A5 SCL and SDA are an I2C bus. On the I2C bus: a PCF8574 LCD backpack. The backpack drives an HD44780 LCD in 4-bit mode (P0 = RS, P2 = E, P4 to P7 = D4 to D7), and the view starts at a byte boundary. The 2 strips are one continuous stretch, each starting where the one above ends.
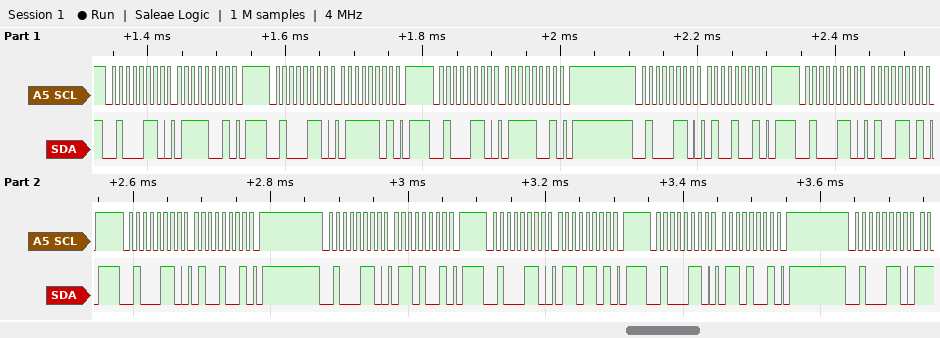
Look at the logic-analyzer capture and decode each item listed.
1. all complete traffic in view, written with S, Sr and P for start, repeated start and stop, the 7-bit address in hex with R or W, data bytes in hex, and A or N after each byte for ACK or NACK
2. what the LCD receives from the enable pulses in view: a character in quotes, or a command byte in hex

S 23W A 79 A P S 23W A 7D A P S 23W A 79 A P S 23W A 49 A P S 23W A 4D A P S 23W A 49 A P S 23W A 69 A P S 23W A 6D A P S 23W A 69 A P S 23W A
't'
